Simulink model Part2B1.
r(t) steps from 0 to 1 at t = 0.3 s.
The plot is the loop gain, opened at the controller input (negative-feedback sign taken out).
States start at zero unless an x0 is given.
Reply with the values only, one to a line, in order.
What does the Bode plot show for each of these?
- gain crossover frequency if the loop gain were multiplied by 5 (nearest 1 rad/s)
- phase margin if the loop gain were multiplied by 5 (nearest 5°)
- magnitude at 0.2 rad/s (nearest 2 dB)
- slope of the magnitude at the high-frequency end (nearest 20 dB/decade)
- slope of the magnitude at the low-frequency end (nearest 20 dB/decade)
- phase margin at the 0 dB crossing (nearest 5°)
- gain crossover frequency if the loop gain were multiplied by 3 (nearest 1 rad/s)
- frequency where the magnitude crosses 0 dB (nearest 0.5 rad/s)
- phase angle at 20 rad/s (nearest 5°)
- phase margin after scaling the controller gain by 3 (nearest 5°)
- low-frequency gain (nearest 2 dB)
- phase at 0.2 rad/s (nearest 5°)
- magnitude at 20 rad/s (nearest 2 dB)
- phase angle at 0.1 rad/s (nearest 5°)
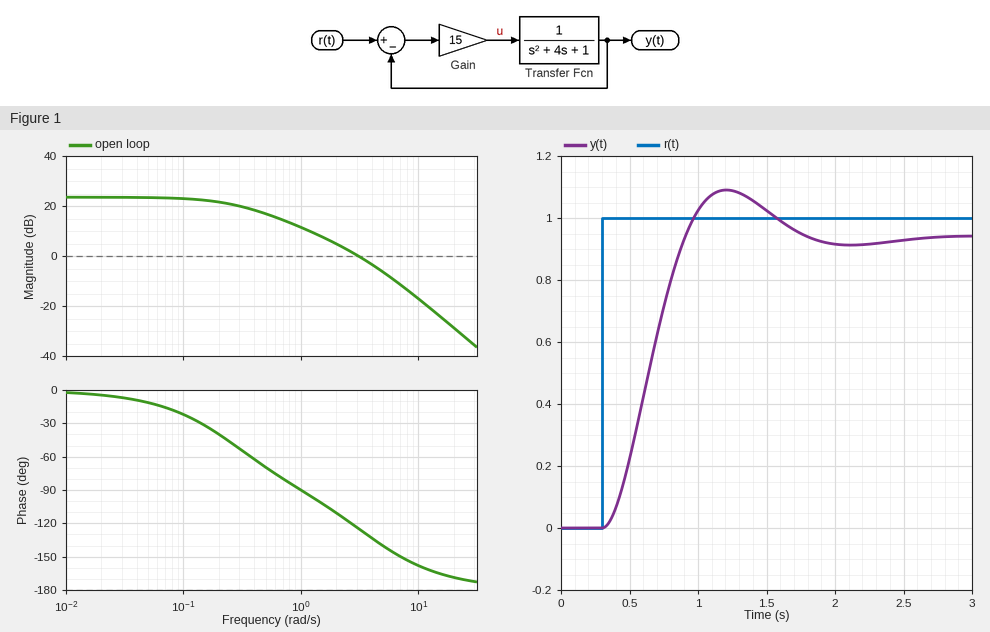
8 rad/s
25°
22 dB
-40 dB/decade
0 dB/decade
55°
6 rad/s
3.0 rad/s
-170°
35°
24 dB
-40°
-28 dB
-20°
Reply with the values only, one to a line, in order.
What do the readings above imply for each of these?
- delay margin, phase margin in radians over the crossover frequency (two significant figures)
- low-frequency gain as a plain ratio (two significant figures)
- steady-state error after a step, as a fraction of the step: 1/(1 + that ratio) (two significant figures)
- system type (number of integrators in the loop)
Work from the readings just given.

0.32 s
16
0.059
0
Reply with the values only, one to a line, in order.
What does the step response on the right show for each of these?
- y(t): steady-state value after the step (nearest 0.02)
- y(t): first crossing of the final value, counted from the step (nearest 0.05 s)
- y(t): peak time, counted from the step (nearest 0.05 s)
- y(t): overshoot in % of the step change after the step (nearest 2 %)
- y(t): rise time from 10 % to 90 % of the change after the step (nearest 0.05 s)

0.94
0.60 s
0.90 s
16 %
0.40 s
